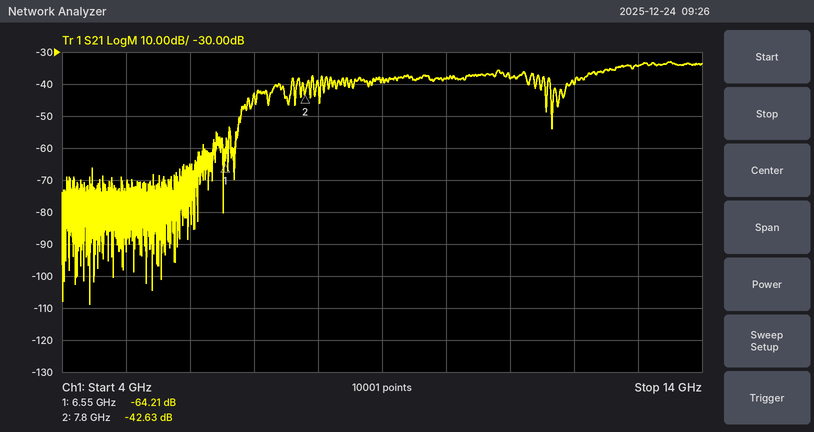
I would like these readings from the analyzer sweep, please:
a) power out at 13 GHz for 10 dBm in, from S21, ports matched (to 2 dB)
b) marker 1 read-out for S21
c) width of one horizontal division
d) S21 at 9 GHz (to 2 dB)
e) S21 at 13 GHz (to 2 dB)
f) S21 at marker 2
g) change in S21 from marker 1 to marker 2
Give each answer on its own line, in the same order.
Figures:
-24 dBm
-64.21 dB
1 GHz
-38 dB
-34 dB
-42.63 dB
21.58 dB
